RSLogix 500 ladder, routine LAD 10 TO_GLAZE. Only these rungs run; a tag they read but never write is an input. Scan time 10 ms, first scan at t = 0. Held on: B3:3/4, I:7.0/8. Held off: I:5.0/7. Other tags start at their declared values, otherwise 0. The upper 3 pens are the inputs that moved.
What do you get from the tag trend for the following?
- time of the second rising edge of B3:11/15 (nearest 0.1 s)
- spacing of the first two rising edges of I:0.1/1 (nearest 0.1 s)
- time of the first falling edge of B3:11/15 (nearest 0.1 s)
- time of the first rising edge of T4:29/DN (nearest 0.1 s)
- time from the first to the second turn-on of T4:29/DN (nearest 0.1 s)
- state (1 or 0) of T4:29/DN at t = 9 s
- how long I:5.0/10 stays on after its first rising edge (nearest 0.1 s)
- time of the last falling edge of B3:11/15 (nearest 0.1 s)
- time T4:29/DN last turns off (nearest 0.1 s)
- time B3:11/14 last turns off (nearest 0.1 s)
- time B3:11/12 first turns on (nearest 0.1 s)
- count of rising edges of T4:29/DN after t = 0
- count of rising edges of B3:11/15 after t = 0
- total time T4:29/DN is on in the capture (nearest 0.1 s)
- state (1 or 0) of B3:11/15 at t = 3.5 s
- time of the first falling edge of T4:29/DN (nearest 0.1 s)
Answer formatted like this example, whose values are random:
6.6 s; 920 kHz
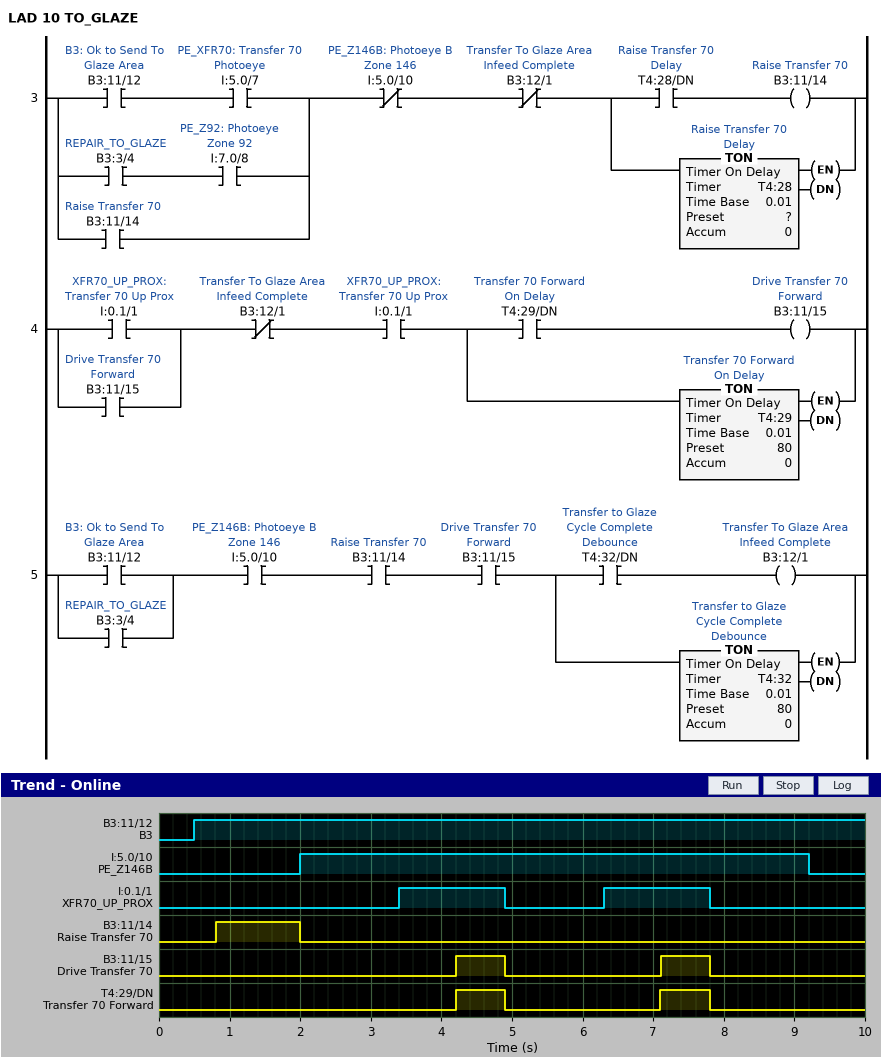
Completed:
7.1 s; 2.9 s; 4.9 s; 4.2 s; 2.9 s; 0; 7.2 s; 7.8 s; 7.8 s; 2.0 s; 0.5 s; 2; 2; 1.4 s; 0; 4.9 s
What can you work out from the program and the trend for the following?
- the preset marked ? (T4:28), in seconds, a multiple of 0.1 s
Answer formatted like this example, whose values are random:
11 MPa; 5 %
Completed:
0.8 s
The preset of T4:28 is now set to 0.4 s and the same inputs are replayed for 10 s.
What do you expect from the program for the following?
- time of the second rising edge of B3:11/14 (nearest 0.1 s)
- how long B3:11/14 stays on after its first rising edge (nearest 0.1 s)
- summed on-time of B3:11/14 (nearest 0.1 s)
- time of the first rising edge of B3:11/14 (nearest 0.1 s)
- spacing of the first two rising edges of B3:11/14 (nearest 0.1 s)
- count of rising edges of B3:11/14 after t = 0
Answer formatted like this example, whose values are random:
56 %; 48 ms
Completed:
9.6 s; 1.6 s; 2.0 s; 0.4 s; 9.2 s; 2
